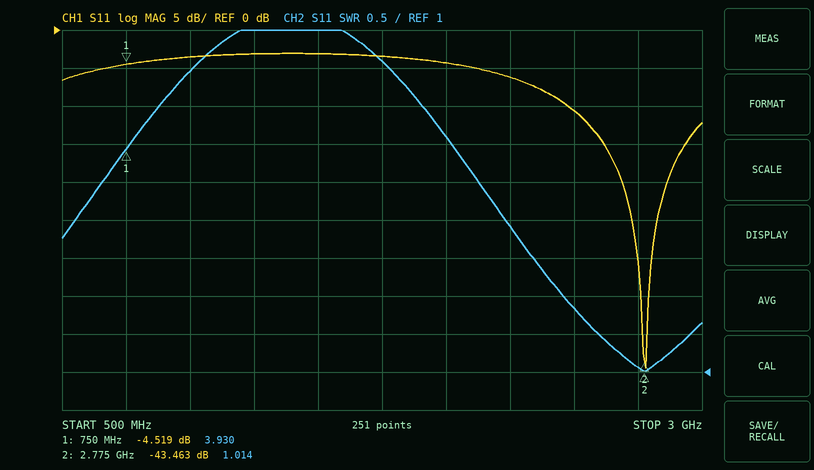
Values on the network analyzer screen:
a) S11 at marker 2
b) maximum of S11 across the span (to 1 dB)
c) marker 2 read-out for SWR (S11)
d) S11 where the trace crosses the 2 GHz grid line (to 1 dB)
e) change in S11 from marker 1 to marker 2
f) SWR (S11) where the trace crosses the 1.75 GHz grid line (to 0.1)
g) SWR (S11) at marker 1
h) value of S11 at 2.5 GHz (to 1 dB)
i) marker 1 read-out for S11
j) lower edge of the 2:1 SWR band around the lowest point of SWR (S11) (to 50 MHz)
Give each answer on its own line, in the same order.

-43.463 dB
-3 dB
1.014
-4 dB
-38.944 dB
5.1
3.930
-11 dB
-4.519 dB
2.45 GHz
